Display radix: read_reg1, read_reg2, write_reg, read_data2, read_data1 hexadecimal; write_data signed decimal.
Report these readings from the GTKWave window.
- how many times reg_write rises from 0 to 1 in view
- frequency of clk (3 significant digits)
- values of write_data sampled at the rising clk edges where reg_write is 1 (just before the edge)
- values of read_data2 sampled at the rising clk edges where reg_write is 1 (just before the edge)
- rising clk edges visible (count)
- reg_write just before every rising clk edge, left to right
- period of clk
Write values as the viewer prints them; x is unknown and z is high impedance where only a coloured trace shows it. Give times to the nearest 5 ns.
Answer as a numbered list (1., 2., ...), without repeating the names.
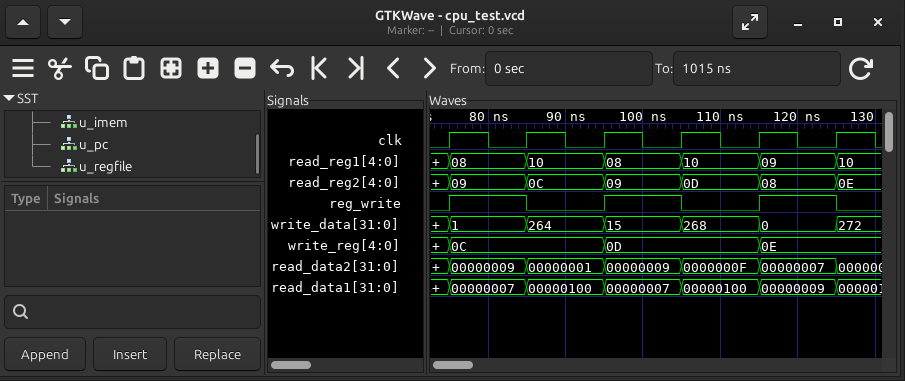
1. 3
2. 100 MHz
3. 1, 15, 0
4. 00000009, 00000009, 00000007
5. 6
6. 0 1 0 1 0 1
7. 10 ns
